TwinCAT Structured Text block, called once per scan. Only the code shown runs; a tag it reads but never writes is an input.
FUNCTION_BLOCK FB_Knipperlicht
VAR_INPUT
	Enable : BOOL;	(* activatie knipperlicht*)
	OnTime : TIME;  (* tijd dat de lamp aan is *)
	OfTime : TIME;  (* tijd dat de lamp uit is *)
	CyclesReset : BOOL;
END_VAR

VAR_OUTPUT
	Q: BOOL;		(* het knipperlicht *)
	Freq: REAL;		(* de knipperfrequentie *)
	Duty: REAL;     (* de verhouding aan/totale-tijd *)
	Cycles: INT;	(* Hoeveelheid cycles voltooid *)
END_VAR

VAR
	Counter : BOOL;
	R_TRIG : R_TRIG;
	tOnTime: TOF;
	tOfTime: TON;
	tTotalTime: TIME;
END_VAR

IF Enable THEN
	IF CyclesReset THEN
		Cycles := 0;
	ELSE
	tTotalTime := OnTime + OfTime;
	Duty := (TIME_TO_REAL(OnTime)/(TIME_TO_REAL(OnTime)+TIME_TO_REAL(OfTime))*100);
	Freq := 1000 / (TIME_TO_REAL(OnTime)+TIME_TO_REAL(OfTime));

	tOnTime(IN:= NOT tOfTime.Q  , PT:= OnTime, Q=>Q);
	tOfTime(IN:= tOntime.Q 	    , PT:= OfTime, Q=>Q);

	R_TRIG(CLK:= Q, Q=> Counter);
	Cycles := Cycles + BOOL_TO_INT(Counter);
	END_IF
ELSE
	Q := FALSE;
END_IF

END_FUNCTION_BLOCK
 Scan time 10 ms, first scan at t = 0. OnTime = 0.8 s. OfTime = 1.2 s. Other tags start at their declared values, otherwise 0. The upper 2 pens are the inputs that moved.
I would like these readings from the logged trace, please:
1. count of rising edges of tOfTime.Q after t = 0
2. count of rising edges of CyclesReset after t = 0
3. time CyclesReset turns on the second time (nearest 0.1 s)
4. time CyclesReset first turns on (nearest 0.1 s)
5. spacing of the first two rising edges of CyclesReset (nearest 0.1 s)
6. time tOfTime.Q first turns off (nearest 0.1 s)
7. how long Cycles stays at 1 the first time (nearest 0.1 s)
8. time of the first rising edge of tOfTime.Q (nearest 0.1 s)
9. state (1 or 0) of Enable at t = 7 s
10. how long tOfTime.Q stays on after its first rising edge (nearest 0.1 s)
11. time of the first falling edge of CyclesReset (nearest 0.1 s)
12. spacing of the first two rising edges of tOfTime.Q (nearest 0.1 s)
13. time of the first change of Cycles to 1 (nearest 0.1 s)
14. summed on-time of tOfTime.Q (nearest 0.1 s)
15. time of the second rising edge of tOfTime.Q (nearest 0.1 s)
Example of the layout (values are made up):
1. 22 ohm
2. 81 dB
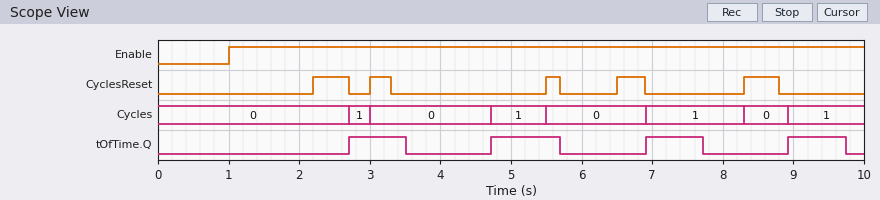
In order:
1. 4
2. 5
3. 3.0 s
4. 2.2 s
5. 0.8 s
6. 3.5 s
7. 0.3 s
8. 2.7 s
9. 1
10. 0.8 s
11. 2.7 s
12. 2.0 s
13. 2.7 s
14. 3.4 s
15. 4.7 s
